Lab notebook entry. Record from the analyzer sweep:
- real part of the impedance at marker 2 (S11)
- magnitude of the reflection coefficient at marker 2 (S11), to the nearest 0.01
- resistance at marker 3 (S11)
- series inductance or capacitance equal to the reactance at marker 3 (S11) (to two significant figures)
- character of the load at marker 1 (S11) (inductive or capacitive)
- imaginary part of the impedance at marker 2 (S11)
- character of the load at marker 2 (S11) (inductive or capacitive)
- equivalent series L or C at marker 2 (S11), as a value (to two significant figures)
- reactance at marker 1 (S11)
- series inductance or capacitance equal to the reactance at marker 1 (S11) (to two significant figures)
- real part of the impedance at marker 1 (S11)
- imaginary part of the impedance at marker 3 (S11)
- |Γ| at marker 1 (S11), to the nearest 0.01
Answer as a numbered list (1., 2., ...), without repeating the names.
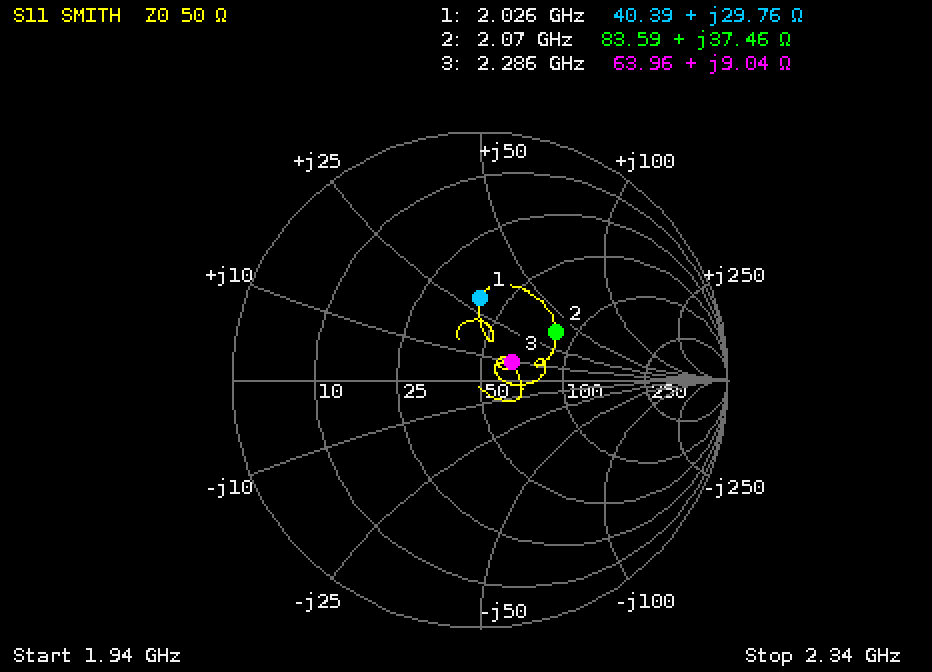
1. 83.59 Ω
2. 0.36
3. 63.96 Ω
4. 630 pH
5. inductive
6. +37.46 Ω
7. inductive
8. 2.9 nH
9. +29.76 Ω
10. 2.3 nH
11. 40.39 Ω
12. +9.04 Ω
13. 0.33
